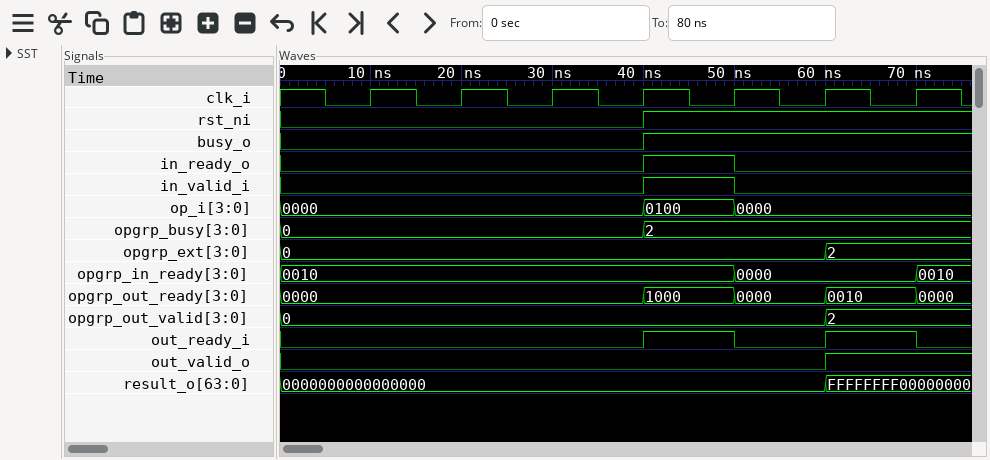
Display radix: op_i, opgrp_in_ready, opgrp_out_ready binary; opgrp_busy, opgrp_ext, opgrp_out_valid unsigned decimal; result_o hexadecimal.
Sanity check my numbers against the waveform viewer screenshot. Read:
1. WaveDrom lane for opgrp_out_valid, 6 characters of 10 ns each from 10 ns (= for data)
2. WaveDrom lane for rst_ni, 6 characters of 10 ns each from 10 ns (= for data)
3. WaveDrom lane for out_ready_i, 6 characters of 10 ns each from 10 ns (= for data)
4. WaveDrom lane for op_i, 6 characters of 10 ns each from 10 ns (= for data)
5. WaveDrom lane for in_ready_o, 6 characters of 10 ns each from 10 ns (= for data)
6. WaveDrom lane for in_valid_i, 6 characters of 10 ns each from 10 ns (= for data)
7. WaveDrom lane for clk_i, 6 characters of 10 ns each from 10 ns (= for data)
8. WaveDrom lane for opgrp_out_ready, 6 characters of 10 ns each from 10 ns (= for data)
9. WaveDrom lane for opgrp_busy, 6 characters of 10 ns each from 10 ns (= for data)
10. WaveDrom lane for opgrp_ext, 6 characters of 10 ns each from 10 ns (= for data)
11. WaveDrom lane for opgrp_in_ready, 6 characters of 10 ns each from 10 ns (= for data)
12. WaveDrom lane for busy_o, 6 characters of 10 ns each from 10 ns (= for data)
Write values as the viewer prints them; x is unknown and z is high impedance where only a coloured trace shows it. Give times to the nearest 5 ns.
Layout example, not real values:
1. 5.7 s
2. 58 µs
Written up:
1. {name: 'opgrp_out_valid', wave: '=....=', data: '0 2'}
2. {name: 'rst_ni', wave: '0..1..'}
3. {name: 'out_ready_i', wave: '0..101'}
4. {name: 'op_i', wave: '=..==.', data: '0000 0100 0000'}
5. {name: 'in_ready_o', wave: '0..10.'}
6. {name: 'in_valid_i', wave: '0..10.'}
7. {name: 'clk_i', wave: 'p.....'}
8. {name: 'opgrp_out_ready', wave: '=..===', data: '0000 1000 0000 0010'}
9. {name: 'opgrp_busy', wave: '=..=..', data: '0 2'}
10. {name: 'opgrp_ext', wave: '=....=', data: '0 2'}
11. {name: 'opgrp_in_ready', wave: '=...=.', data: '0010 0000'}
12. {name: 'busy_o', wave: '0..1..'}
